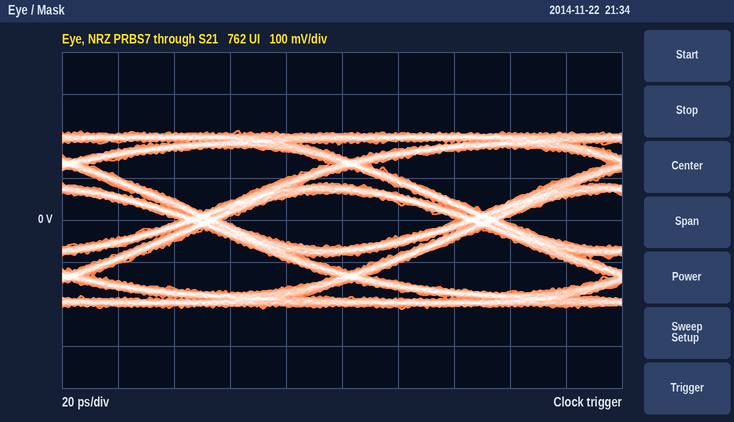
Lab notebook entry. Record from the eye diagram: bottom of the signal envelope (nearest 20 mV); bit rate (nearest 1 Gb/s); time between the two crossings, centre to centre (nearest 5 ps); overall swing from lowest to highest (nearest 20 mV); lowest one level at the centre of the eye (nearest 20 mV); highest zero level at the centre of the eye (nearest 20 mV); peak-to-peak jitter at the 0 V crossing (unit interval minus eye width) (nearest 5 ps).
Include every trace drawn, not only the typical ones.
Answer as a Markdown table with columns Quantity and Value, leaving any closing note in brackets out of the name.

| Quantity | Value |
|---|---|
| bottom of the signal envelope | -220 mV |
| bit rate | 10 Gb/s |
| time between the two crossings, centre to centre | 100 ps |
| overall swing from lowest to highest | 420 mV |
| lowest one level at the centre of the eye | 60 mV |
| highest zero level at the centre of the eye | -60 mV |
| peak-to-peak jitter at the 0 V crossing (unit interval minus eye width) | 15 ps |
